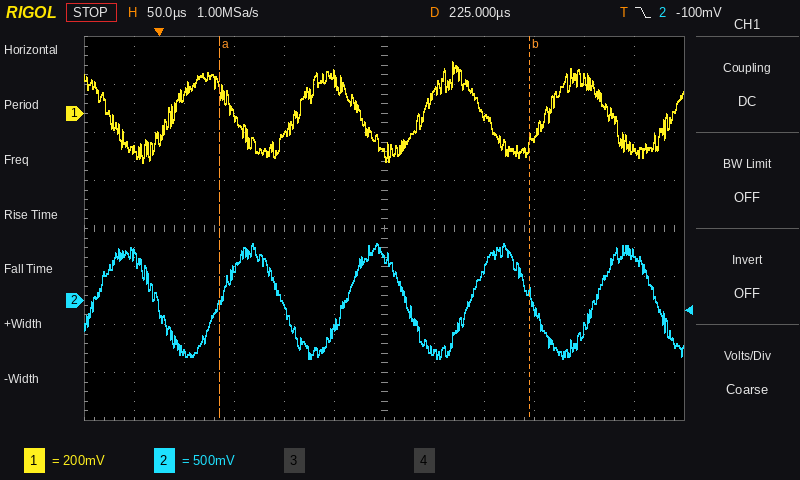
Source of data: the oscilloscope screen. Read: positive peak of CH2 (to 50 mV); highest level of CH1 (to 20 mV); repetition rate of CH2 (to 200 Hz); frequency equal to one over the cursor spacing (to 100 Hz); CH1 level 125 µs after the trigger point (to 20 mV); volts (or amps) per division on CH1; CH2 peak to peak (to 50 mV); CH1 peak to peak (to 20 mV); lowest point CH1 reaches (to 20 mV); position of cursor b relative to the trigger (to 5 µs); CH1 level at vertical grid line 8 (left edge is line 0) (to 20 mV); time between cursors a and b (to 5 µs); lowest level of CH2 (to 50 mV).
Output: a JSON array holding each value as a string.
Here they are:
["600 mV", "220 mV", "8.0 kHz", "3.2 kHz", "-80 mV", "200 mV", "1.20 V", "420 mV", "-200 mV", "+370 µs", "0 mV", "310 µs", "-600 mV"]
